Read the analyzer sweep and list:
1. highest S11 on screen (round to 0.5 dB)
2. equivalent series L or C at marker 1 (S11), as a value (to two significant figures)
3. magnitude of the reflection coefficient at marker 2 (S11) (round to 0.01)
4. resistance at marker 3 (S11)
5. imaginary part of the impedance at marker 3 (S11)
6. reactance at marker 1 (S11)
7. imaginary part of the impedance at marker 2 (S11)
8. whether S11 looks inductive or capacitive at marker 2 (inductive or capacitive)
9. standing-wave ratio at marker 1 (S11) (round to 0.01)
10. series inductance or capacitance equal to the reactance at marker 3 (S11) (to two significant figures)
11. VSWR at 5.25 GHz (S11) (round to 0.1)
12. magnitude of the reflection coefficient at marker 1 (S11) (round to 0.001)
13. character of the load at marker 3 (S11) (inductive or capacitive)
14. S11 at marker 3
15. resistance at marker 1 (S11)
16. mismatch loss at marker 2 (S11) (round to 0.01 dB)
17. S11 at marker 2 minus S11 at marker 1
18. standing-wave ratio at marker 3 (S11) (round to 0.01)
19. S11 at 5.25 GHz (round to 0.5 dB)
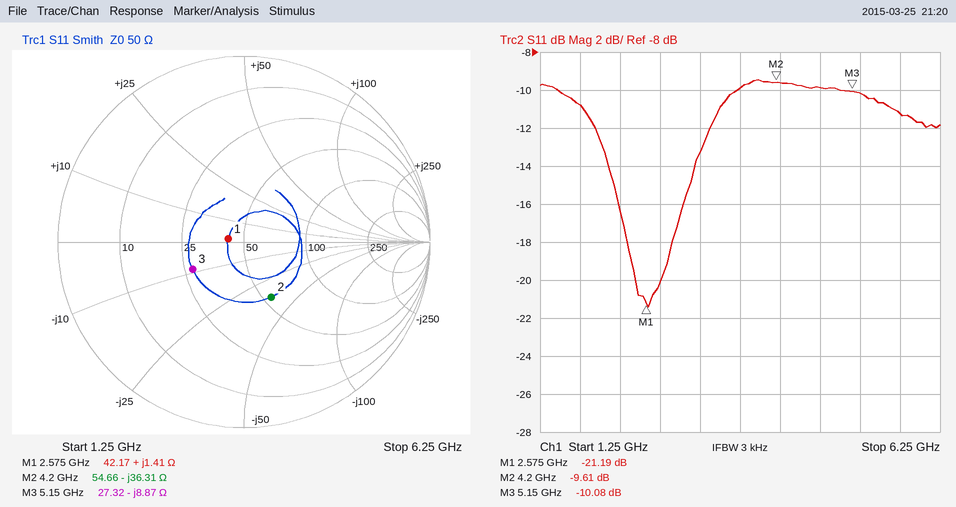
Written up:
-9.5 dB
87 pH
0.33
27.32 Ω
-8.87 Ω
+1.41 Ω
-36.31 Ω
capacitive
1.19
3.5 pF
1.9
0.087
capacitive
-10.08 dB
42.17 Ω
0.50 dB
11.58 dB
1.91
-10.0 dB
